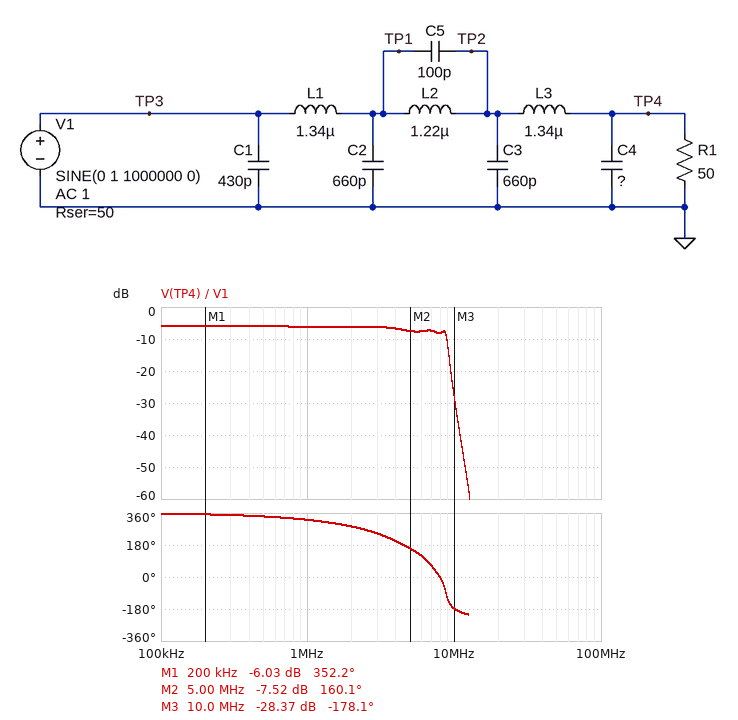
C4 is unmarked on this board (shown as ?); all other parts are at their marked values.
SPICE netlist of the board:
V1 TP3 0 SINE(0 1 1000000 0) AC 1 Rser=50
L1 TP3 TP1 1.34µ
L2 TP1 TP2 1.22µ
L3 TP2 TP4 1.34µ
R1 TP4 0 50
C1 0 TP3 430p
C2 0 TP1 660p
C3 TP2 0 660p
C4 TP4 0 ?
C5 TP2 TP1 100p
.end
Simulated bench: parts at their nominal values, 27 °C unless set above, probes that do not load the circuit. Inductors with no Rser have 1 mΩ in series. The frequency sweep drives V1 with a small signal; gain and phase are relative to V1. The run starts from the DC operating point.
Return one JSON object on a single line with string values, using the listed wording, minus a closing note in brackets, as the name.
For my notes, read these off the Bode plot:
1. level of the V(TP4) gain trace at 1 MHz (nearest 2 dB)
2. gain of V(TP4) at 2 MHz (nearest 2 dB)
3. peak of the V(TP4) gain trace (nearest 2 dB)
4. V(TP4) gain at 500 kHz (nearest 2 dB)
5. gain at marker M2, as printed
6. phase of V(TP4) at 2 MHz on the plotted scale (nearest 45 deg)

{"level of the V(TP4) gain trace at 1 MHz": "-6 dB", "gain of V(TP4) at 2 MHz": "-6 dB", "peak of the V(TP4) gain trace": "-6 dB", "V(TP4) gain at 500 kHz": "-6 dB", "gain at marker M2, as printed": "-7.52 dB", "phase of V(TP4) at 2 MHz on the plotted scale": "270 deg"}
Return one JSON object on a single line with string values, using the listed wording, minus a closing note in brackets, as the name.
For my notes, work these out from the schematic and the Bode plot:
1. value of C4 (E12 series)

{"value of C4": "1 nF"}
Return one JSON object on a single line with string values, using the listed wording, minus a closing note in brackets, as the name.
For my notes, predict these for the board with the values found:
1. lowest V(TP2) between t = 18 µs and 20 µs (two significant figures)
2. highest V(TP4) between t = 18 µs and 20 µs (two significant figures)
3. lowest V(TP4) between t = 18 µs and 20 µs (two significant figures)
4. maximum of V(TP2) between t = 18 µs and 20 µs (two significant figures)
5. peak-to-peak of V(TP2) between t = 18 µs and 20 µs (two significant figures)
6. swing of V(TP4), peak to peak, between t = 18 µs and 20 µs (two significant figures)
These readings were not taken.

{"lowest V(TP2) between t = 18 µs and 20 µs": "-470 mV", "highest V(TP4) between t = 18 µs and 20 µs": "490 mV", "lowest V(TP4) between t = 18 µs and 20 µs": "-490 mV", "maximum of V(TP2) between t = 18 µs and 20 µs": "470 mV", "peak-to-peak of V(TP2) between t = 18 µs and 20 µs": "950 mV", "swing of V(TP4), peak to peak, between t = 18 µs and 20 µs": "990 mV"}
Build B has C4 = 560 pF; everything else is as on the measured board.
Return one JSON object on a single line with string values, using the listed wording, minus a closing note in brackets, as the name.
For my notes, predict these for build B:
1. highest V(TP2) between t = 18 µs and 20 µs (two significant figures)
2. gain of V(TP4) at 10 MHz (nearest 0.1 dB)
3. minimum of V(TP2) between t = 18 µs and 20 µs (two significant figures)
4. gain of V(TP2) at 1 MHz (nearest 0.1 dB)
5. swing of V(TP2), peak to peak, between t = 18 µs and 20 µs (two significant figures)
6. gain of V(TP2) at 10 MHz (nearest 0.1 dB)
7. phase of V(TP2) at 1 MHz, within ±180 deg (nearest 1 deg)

{"highest V(TP2) between t = 18 µs and 20 µs": "490 mV", "gain of V(TP4) at 10 MHz": "-23.0 dB", "minimum of V(TP2) between t = 18 µs and 20 µs": "-490 mV", "gain of V(TP2) at 1 MHz": "-6.2 dB", "swing of V(TP2), peak to peak, between t = 18 µs and 20 µs": "980 mV", "gain of V(TP2) at 10 MHz": "-14.7 dB", "phase of V(TP2) at 1 MHz, within ±180 deg": "-25 deg"}
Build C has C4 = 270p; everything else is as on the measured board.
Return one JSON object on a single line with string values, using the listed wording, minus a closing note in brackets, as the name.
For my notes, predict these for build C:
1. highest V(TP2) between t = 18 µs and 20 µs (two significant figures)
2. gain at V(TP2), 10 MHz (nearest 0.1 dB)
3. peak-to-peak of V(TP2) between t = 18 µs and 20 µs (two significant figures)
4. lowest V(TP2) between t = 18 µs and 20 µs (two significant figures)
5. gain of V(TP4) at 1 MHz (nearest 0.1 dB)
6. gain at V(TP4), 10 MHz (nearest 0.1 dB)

{"highest V(TP2) between t = 18 µs and 20 µs": "500 mV", "gain at V(TP2), 10 MHz": "-16.0 dB", "peak-to-peak of V(TP2) between t = 18 µs and 20 µs": "1.0 V", "lowest V(TP2) between t = 18 µs and 20 µs": "-500 mV", "gain of V(TP4) at 1 MHz": "-6.0 dB", "gain at V(TP4), 10 MHz": "-20.8 dB"}
